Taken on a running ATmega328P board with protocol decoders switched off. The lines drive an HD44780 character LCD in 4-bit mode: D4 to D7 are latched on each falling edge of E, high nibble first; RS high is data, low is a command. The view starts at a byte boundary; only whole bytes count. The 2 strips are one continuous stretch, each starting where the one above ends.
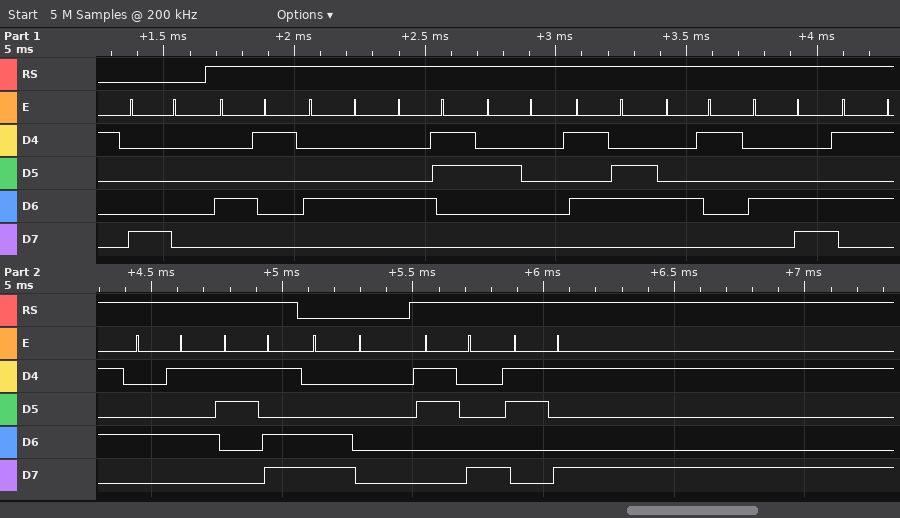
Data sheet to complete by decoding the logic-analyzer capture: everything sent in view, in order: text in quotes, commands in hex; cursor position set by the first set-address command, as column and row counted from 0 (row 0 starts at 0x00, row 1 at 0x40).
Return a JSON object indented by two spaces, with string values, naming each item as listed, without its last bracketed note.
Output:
{
  "everything sent in view, in order: text in quotes, commands in hex": "0x80 \"ADC VALUE=\" 0xC0 \"89\"",
  "cursor position set by the first set-address command, as column and row counted from 0": "column 0, row 0"
}
